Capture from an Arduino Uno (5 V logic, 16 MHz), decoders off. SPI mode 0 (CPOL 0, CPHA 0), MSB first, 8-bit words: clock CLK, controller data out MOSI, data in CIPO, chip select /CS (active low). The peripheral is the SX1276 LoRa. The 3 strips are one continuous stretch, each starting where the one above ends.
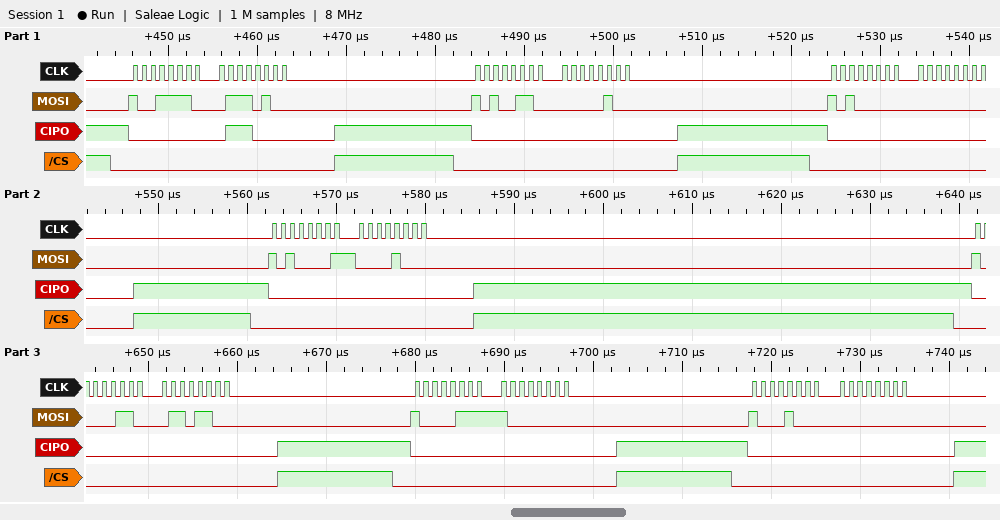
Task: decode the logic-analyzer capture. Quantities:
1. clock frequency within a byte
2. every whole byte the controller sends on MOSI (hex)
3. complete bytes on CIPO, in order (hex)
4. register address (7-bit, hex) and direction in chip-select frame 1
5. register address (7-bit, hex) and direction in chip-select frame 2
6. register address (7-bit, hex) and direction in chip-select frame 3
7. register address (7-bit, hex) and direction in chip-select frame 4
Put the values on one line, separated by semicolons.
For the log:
1 MHz; 0x9E 0x74 0xA6 0x04 0xA0 0x00 0xA1 0x08 0x86 0x6C 0x87 0x80 0x88 0x00; 0x00 0x70 0x00 0x00 0x00 0x00 0x00 0x00 0x00 0x00 0x00 0x00 0x00 0x00; 0x1E write; 0x26 write; 0x20 write; 0x21 write
